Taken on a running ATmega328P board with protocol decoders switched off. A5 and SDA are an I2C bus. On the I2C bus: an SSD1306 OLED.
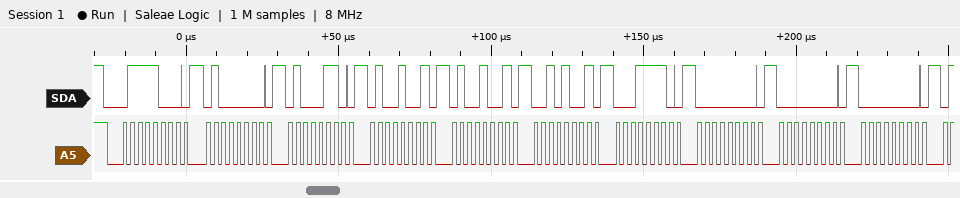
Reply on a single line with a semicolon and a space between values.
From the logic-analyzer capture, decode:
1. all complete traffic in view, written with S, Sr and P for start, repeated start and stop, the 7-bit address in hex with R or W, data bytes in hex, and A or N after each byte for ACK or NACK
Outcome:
S 3CW A 40 A 46 A 49 A 49 A 29 A 1E A 00 A 00 A 00 A
